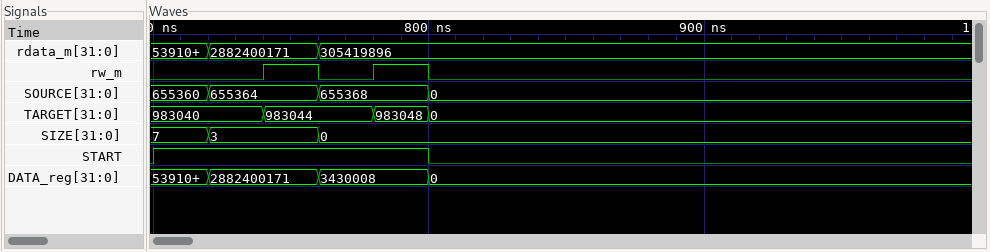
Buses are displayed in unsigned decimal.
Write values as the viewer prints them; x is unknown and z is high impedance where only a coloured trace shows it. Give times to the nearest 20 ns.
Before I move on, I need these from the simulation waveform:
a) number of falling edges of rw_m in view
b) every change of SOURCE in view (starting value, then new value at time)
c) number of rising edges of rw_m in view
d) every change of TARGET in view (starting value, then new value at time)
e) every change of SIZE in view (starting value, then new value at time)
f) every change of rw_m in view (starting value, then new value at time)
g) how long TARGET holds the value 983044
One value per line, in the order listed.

2
655360, 655364 at 720 ns, 655368 at 760 ns, 0 at 800 ns
2
983040, 983044 at 740 ns, 983048 at 780 ns, 0 at 800 ns
7, 3 at 720 ns, 0 at 760 ns
0, 1 at 740 ns, 0 at 760 ns, 1 at 780 ns, 0 at 800 ns
40 ns
